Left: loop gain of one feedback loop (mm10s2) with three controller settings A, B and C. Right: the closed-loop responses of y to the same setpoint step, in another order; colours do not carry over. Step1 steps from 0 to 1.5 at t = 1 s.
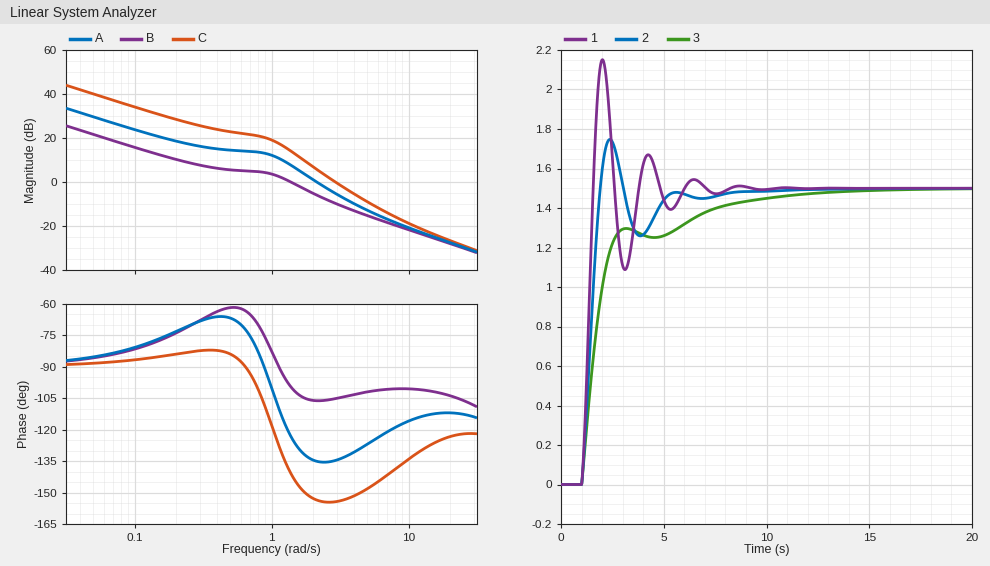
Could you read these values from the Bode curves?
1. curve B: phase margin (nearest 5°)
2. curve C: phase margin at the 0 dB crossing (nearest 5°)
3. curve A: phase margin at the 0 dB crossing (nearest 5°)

80°
25°
45°
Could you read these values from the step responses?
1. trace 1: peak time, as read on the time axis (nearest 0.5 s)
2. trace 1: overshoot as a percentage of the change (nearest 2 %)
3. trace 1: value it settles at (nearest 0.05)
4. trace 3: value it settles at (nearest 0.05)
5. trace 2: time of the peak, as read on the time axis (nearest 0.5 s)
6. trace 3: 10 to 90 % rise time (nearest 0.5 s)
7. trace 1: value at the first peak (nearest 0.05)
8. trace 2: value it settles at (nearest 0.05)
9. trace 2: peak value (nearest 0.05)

2.0 s
44 %
1.50
1.50
2.5 s
5.5 s
2.15
1.50
1.75
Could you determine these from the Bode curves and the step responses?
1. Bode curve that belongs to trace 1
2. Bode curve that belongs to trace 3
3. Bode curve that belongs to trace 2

C
B
A
